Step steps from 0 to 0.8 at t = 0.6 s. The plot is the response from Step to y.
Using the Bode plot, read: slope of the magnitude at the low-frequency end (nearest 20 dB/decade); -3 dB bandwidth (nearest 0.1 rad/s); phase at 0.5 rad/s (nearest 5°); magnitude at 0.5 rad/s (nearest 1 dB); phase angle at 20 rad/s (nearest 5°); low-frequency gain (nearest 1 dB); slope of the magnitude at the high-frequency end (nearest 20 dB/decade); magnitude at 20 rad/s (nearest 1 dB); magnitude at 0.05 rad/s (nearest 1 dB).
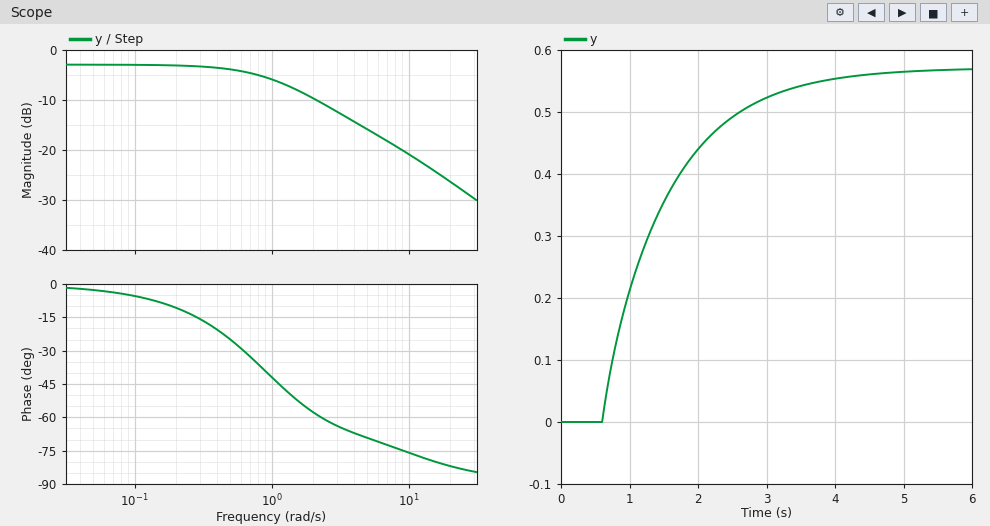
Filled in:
0 dB/decade
1.0 rad/s
-25°
-4 dB
-80°
-3 dB
-20 dB/decade
-26 dB
-3 dB
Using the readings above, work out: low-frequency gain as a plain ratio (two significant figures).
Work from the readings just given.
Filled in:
0.71
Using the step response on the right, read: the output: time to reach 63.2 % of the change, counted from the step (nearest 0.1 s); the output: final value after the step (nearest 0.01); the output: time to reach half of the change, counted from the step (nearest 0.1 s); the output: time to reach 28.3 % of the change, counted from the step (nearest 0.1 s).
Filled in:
0.9 s
0.57
0.6 s
0.3 s
